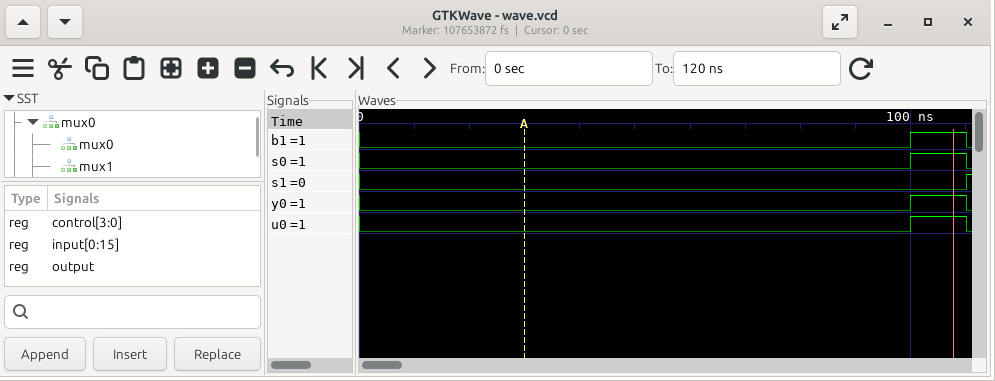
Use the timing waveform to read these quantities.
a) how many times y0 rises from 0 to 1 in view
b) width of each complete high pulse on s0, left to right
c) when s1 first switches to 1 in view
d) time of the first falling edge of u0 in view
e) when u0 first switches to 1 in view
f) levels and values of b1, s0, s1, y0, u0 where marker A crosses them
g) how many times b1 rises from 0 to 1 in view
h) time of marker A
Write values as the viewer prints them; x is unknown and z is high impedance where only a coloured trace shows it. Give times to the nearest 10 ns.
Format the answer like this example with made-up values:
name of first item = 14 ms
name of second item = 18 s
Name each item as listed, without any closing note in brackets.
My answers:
how many times y0 rises from 0 to 1 in view = 1
width of each complete high pulse on s0, left to right = 10 ns
when s1 first switches to 1 in view = 110 ns
time of the first falling edge of u0 in view = 110 ns
when u0 first switches to 1 in view = 100 ns
levels and values of b1, s0, s1, y0, u0 where marker A crosses them = b1=0, s0=0, s1=0, y0=0, u0=0
how many times b1 rises from 0 to 1 in view = 1
time of marker A = 30 ns
